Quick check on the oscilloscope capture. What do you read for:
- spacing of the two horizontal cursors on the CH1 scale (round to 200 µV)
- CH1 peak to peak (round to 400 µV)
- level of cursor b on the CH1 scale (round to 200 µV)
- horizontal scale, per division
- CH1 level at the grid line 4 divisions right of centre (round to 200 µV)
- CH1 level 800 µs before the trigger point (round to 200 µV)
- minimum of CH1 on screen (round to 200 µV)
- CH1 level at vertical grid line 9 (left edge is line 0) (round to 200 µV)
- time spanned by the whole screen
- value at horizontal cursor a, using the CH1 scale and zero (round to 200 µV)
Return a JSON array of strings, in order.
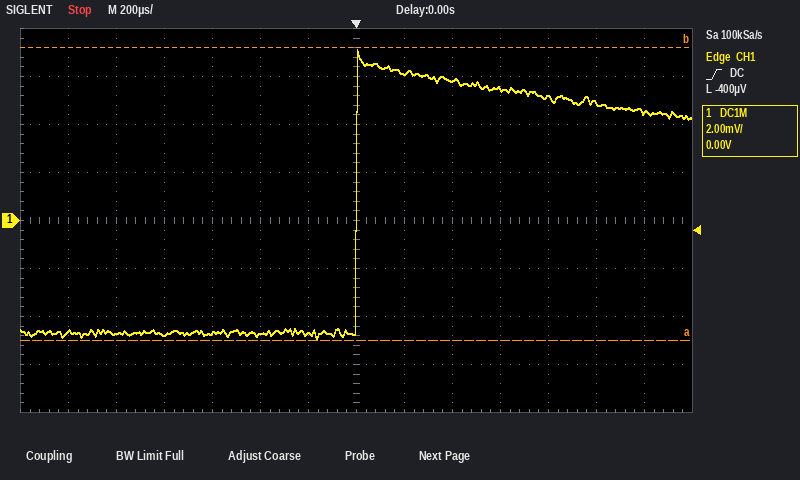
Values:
["12.2 mV", "12.0 mV", "7.2 mV", "200 µs", "5.2 mV", "-4.8 mV", "-5.0 mV", "5.8 mV", "2.8 ms", "-5.0 mV"]
